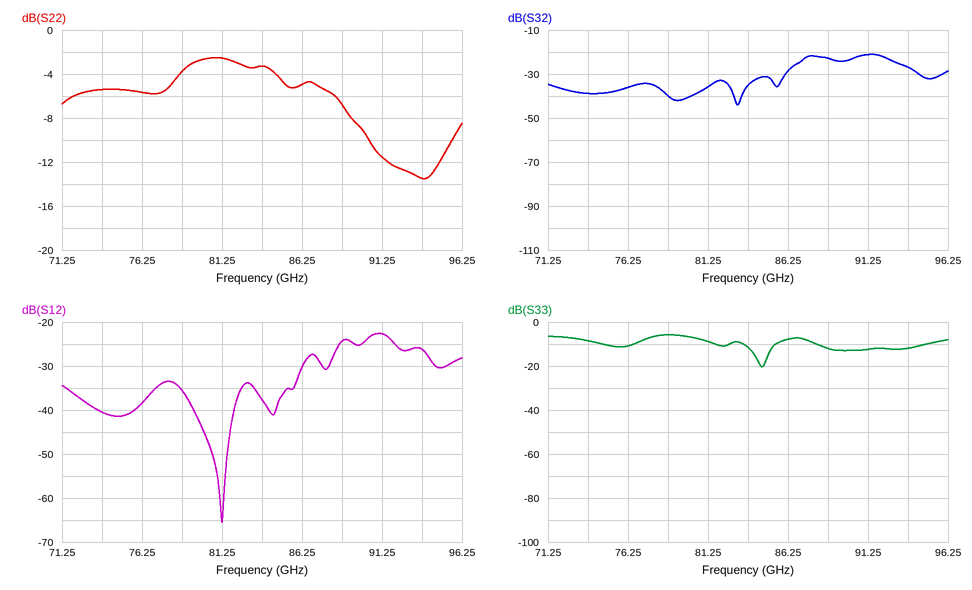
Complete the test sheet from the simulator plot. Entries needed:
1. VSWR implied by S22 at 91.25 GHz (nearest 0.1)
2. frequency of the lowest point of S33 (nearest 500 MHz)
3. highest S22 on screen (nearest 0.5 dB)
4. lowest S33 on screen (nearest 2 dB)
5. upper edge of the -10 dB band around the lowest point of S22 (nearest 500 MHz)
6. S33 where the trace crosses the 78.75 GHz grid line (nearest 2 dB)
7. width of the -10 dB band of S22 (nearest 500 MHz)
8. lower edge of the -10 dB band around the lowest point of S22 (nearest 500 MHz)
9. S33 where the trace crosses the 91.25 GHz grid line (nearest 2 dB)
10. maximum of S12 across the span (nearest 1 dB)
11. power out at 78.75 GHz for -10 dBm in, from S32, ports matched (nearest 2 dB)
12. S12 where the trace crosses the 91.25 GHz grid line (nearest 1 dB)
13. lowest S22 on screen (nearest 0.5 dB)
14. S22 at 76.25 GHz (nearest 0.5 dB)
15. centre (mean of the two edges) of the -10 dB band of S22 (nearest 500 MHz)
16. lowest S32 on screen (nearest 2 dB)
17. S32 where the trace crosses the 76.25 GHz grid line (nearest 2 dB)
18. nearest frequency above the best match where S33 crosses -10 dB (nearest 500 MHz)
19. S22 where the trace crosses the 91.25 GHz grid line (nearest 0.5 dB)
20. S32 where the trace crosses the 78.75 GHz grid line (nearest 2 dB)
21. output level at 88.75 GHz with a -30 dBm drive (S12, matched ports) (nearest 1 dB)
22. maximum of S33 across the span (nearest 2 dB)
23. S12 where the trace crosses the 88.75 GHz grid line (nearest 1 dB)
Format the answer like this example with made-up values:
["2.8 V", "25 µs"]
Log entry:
["1.7", "84.5 GHz", "-2.5 dB", "-20 dB", "95.5 GHz", "-6 dB", "5.0 GHz", "90.5 GHz", "-12 dB", "-23 dB", "-50 dBm", "-23 dB", "-13.5 dB", "-5.5 dB", "93.0 GHz", "-44 dB", "-36 dB", "85.5 GHz", "-11.5 dB", "-40 dB", "-54 dBm", "-6 dB", "-24 dB"]
